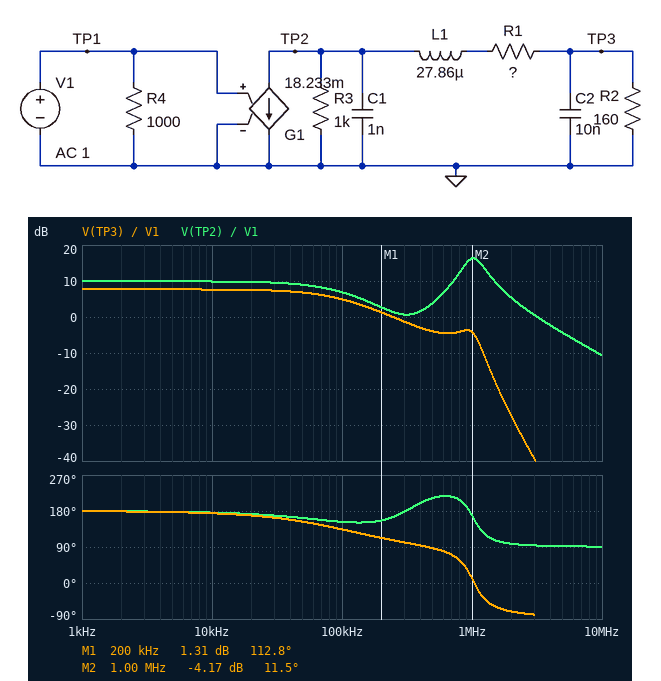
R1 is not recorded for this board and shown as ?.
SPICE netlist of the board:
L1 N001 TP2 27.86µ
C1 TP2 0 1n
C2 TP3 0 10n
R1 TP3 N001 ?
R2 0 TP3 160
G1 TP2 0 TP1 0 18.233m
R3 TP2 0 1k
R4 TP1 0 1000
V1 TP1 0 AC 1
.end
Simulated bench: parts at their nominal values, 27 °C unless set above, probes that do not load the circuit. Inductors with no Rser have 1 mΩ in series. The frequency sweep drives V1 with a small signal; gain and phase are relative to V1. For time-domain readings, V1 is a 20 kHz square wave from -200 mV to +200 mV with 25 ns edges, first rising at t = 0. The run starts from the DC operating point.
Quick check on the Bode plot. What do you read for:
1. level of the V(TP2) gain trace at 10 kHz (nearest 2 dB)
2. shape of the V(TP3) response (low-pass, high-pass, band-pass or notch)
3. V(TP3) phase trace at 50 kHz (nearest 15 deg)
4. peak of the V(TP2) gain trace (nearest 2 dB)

10 dB
low-pass
150 deg
16 dB
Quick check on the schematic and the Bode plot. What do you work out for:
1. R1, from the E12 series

47 Ω
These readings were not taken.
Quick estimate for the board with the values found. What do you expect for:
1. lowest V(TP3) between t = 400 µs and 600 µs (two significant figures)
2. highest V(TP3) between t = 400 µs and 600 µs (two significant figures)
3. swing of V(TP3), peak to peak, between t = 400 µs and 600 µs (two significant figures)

-480 mV
480 mV
970 mV
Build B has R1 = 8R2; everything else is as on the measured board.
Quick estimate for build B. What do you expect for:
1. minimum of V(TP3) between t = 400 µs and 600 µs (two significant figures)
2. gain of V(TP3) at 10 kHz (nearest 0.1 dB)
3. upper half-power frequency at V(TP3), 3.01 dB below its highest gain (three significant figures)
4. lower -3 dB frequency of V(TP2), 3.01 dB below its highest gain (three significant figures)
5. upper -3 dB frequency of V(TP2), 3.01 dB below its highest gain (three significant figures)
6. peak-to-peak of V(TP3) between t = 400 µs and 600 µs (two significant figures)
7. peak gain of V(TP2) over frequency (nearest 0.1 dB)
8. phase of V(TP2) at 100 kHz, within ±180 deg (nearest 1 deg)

-500 mV
7.9 dB
107 kHz
912 kHz
1.11 MHz
1.0 V
22.4 dB
145 deg
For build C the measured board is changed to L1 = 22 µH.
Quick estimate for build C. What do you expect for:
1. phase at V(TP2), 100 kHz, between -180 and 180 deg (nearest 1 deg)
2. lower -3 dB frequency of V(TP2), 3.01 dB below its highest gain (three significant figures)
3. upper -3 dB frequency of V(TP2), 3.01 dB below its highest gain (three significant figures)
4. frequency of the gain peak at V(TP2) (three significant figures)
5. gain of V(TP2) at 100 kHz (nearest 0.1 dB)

152 deg
934 kHz
1.43 MHz
1.15 MHz
7.0 dB
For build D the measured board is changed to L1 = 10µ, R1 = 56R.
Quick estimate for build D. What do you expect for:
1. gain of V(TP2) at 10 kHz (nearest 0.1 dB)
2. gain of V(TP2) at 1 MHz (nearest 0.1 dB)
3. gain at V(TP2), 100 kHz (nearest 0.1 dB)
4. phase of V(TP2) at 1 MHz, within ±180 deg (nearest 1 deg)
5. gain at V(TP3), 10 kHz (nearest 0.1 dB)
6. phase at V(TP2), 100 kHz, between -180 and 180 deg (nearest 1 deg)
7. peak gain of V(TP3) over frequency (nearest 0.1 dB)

10.2 dB
3.9 dB
7.5 dB
-169 deg
7.6 dB
151 deg
7.6 dB
